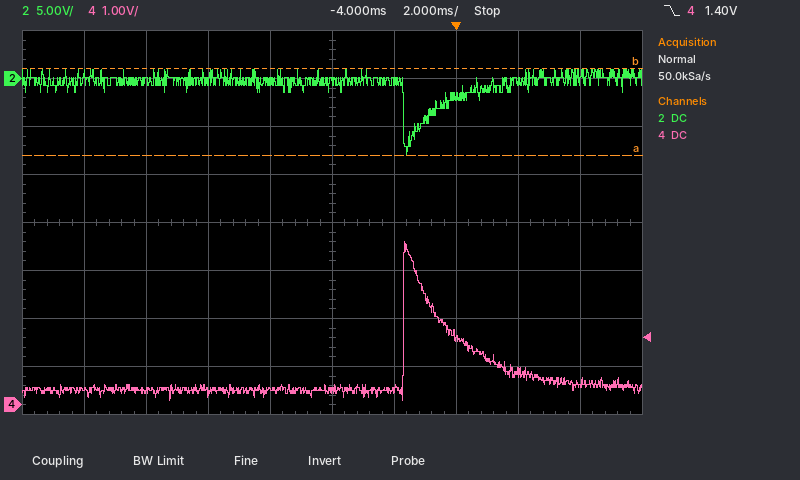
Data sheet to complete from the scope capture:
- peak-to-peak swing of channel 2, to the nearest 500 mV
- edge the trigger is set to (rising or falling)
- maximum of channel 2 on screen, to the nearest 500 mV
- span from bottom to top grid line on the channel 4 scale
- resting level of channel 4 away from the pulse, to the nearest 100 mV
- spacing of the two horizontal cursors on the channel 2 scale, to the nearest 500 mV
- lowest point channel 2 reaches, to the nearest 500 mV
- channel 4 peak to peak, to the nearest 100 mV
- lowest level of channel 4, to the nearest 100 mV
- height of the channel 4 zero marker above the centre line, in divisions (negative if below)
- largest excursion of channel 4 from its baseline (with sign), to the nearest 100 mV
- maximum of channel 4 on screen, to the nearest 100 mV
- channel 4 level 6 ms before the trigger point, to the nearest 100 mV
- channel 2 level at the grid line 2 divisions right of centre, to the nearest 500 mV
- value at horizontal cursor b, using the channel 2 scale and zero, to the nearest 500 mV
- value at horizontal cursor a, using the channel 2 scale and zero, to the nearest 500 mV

9.0 V
falling
1.0 V
8 V
300 mV
9.0 V
-8.0 V
3.3 V
100 mV
-3.8 div
+3.1 V
3.4 V
300 mV
-2.0 V
1.0 V
-8.0 V
